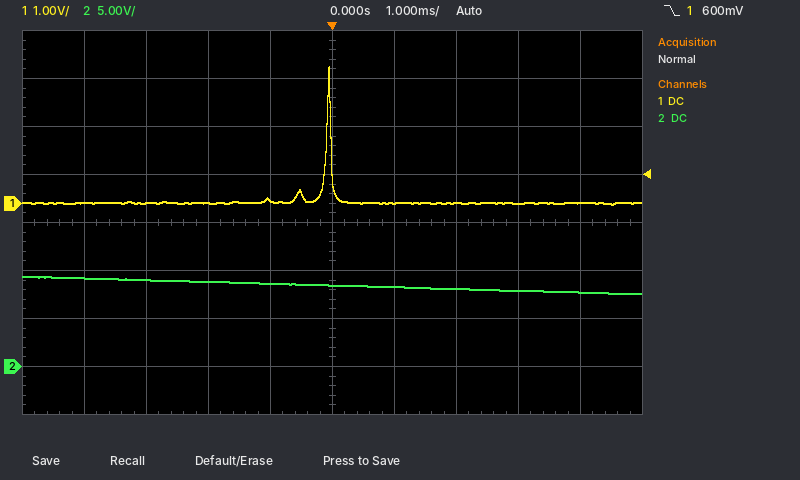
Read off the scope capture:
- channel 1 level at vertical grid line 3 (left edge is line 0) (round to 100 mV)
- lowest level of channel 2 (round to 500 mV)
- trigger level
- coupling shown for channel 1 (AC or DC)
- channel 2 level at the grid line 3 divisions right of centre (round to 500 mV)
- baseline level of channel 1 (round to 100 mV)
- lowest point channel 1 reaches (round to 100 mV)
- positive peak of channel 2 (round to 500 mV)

0.0 V
7.5 V
600 mV
DC
8.0 V
0.0 V
0.0 V
9.5 V
